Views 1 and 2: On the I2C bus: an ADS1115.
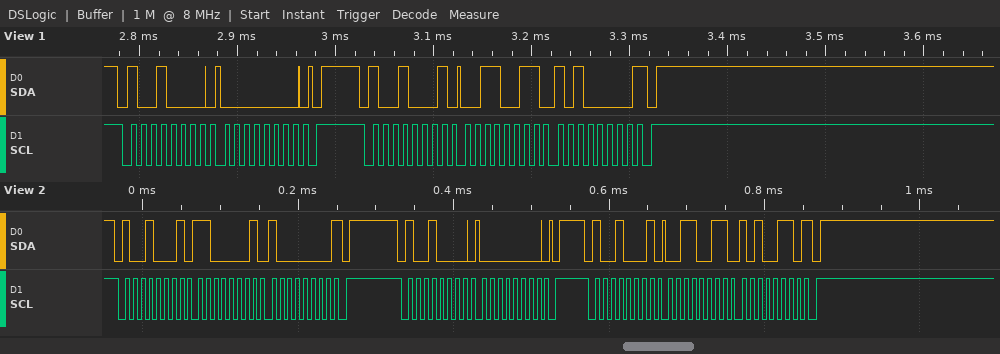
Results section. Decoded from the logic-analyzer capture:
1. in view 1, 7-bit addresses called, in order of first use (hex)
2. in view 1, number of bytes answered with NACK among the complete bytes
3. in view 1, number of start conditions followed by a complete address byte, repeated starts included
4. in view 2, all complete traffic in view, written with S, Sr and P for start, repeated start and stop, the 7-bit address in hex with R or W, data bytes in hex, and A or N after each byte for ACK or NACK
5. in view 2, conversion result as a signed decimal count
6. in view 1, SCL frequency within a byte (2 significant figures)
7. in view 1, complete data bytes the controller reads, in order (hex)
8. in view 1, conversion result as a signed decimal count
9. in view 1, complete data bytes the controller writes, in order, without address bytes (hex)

0x48
1
2
S 48R A C1 A 80 N P S 48W A 00 A P S 48R A 33 A A6 N P
13222
100 kHz
33 A0
13216
00
